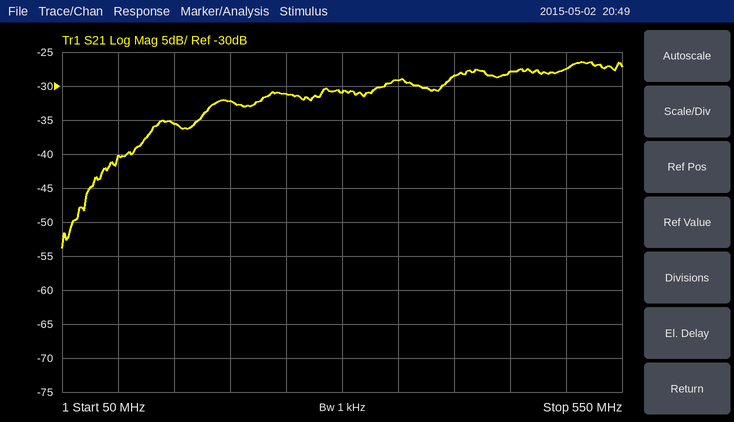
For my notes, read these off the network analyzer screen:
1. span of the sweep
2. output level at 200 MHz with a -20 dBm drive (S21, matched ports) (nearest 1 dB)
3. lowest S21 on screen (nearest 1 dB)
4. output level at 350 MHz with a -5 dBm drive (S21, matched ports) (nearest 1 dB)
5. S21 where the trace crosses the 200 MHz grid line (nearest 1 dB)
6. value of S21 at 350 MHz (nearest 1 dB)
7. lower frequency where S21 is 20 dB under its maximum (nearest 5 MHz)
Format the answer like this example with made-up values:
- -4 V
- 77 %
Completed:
- 500 MHz
- -52 dBm
- -54 dB
- -34 dBm
- -32 dB
- -29 dB
- 70 MHz
